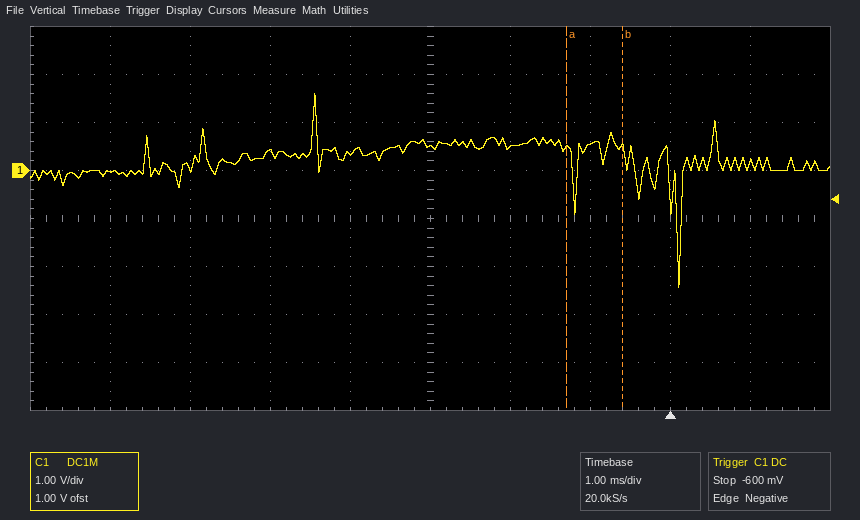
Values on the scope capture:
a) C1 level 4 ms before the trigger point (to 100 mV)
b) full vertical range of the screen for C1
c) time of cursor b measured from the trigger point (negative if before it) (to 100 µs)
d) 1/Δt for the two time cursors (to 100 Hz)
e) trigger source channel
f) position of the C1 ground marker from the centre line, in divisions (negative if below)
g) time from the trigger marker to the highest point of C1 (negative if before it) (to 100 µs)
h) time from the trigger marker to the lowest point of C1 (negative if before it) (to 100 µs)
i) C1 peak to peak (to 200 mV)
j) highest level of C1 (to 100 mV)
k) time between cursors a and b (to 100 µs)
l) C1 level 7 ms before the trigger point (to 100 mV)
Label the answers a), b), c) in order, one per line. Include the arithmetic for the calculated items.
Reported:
a) 400 mV
b) 8 V
c) -600 µs
d) 1 / 700 µs ≈ 1.4 kHz
e) C1
f) +1.0 div
g) -4.4 ms
h) +100 µs
i) 4.0 V
j) 1.6 V
k) 700 µs
l) 0.0 V
